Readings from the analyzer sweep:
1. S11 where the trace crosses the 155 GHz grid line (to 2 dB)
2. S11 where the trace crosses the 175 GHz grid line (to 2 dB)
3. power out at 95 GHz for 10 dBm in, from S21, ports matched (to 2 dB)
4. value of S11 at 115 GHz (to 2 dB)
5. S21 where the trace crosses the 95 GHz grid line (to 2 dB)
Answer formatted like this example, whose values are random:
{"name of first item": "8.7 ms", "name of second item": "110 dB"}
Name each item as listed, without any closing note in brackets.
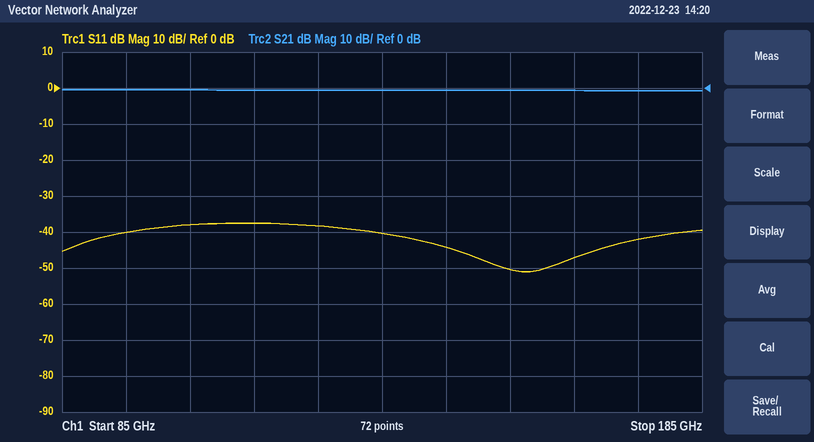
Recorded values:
{"S11 where the trace crosses the 155 GHz grid line": "-50 dB", "S11 where the trace crosses the 175 GHz grid line": "-42 dB", "power out at 95 GHz for 10 dBm in, from S21, ports matched": "10 dBm", "value of S11 at 115 GHz": "-38 dB", "S21 where the trace crosses the 95 GHz grid line": "0 dB"}
